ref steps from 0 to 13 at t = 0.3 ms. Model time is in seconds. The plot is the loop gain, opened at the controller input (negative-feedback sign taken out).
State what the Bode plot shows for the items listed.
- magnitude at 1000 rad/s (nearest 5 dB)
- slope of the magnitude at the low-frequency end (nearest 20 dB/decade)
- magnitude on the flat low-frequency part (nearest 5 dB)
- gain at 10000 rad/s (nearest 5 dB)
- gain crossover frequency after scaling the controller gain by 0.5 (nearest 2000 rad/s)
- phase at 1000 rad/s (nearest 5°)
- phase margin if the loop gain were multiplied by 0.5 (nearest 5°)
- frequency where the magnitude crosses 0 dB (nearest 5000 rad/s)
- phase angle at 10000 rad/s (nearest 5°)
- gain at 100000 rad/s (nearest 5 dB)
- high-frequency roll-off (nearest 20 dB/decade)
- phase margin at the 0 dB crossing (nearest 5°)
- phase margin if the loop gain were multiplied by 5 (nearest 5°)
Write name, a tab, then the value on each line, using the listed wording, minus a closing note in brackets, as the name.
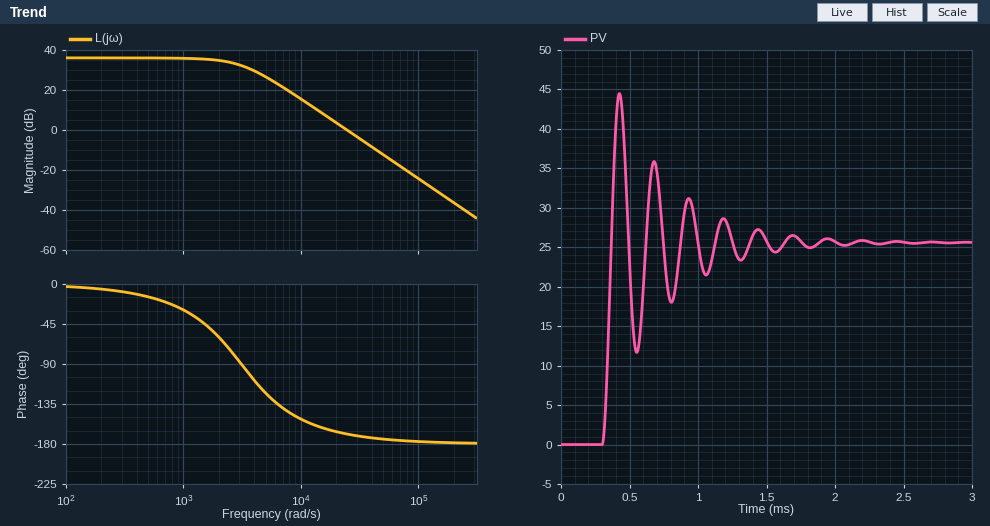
magnitude at 1000 rad/s	35 dB
slope of the magnitude at the low-frequency end	0 dB/decade
magnitude on the flat low-frequency part	35 dB
gain at 10000 rad/s	15 dB
gain crossover frequency after scaling the controller gain by 0.5	18000 rad/s
phase at 1000 rad/s	-30°
phase margin if the loop gain were multiplied by 0.5	15°
frequency where the magnitude crosses 0 dB	25000 rad/s
phase angle at 10000 rad/s	-150°
gain at 100000 rad/s	-25 dB
high-frequency roll-off	-40 dB/decade
phase margin at the 0 dB crossing	10°
phase margin if the loop gain were multiplied by 5	5°
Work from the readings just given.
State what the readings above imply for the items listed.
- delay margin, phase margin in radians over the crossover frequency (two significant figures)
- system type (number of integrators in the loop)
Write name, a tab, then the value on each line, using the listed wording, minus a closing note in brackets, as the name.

delay margin, phase margin in radians over the crossover frequency	0.0000070 s
system type	0
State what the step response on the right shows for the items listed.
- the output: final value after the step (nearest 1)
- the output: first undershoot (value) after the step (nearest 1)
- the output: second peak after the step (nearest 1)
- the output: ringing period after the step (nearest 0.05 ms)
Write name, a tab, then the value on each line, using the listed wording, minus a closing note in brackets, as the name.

the output: final value after the step	26
the output: first undershoot (value) after the step	12
the output: second peak after the step	36
the output: ringing period after the step	0.25 ms
